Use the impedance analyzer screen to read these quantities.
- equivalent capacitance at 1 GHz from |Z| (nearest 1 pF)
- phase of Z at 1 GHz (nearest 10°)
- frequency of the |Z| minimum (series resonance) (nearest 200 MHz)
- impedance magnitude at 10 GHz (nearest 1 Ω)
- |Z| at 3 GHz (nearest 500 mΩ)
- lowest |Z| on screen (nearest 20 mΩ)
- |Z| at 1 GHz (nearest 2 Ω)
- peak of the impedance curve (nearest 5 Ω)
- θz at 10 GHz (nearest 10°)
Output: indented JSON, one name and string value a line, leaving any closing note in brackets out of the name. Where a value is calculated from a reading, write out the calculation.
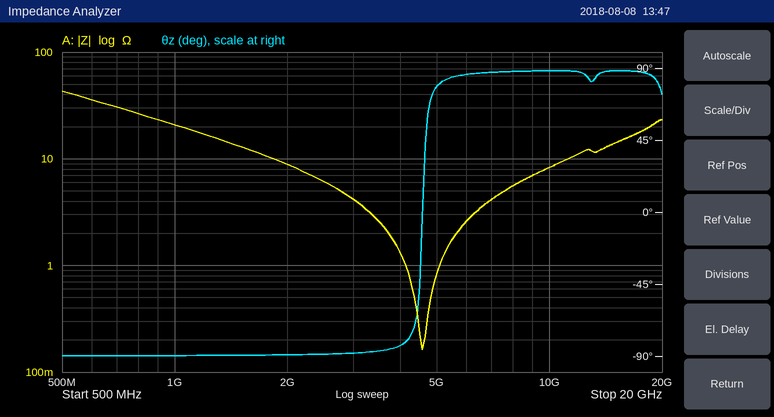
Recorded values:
{
  "equivalent capacitance at 1 GHz from |Z|": "C = 1/(2π × 1 GHz × 20 Ω) ≈ 8 pF",
  "phase of Z at 1 GHz": "-90°",
  "frequency of the |Z| minimum (series resonance)": "4.6 GHz",
  "impedance magnitude at 10 GHz": "8 Ω",
  "|Z| at 3 GHz": "4.0 Ω",
  "lowest |Z| on screen": "160 mΩ",
  "|Z| at 1 GHz": "20 Ω",
  "peak of the impedance curve": "45 Ω",
  "θz at 10 GHz": "90°"
}
